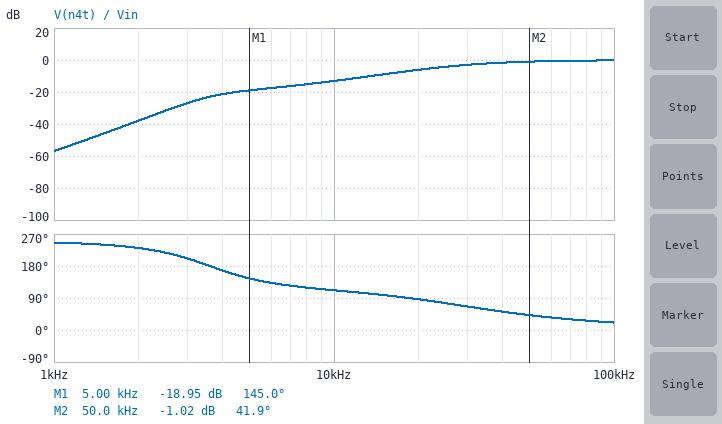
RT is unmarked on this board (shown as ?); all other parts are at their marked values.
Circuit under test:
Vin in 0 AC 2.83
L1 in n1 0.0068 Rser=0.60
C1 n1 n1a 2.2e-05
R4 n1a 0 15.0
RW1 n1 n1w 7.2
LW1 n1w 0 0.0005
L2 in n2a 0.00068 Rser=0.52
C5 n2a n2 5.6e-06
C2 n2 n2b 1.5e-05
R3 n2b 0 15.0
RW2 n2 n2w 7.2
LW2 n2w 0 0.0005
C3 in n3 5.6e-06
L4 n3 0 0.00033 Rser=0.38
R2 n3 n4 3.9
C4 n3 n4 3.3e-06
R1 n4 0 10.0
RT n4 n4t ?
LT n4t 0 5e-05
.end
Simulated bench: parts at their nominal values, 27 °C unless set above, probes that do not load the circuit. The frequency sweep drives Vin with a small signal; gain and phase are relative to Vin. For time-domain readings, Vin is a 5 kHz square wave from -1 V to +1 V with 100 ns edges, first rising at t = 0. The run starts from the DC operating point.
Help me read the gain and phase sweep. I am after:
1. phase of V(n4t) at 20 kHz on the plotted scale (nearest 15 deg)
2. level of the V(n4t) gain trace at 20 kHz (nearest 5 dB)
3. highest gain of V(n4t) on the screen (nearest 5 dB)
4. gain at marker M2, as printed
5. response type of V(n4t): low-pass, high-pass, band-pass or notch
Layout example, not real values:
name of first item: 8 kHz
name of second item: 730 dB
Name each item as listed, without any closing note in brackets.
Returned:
phase of V(n4t) at 20 kHz on the plotted scale: 90 deg
level of the V(n4t) gain trace at 20 kHz: -5 dB
highest gain of V(n4t) on the screen: 0 dB
gain at marker M2, as printed: -1.02 dB
response type of V(n4t): low-pass, high-pass, band-pass or notch: high-pass
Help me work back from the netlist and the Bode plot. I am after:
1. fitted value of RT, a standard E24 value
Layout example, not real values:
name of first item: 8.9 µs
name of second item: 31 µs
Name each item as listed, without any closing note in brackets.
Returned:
fitted value of RT, a standard E24 value: 9.1 Ω
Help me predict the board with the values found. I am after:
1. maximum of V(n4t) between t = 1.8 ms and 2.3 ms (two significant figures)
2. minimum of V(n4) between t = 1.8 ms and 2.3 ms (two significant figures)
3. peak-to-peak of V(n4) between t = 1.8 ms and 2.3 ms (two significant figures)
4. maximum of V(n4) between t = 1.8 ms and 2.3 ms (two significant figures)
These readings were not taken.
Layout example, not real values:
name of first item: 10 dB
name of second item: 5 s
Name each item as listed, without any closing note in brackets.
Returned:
maximum of V(n4t) between t = 1.8 ms and 2.3 ms: 2.0 V
minimum of V(n4) between t = 1.8 ms and 2.3 ms: -2.3 V
peak-to-peak of V(n4) between t = 1.8 ms and 2.3 ms: 4.5 V
maximum of V(n4) between t = 1.8 ms and 2.3 ms: 2.3 V
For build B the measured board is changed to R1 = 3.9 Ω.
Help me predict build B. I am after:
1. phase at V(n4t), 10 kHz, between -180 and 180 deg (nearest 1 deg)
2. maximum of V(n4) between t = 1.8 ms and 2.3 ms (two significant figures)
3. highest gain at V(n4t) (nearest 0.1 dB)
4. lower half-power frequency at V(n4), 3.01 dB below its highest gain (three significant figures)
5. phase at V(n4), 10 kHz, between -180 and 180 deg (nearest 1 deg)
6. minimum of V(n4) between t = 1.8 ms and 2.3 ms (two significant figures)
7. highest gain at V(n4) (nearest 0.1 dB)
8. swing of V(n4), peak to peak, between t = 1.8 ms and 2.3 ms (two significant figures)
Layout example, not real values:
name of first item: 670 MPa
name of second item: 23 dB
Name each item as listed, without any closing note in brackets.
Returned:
phase at V(n4t), 10 kHz, between -180 and 180 deg: 120 deg
maximum of V(n4) between t = 1.8 ms and 2.3 ms: 2.1 V
highest gain at V(n4t): 0 dB
lower half-power frequency at V(n4), 3.01 dB below its highest gain: 24.3 kHz
phase at V(n4), 10 kHz, between -180 and 180 deg: 49 deg
minimum of V(n4) between t = 1.8 ms and 2.3 ms: -2.1 V
highest gain at V(n4): 0 dB
swing of V(n4), peak to peak, between t = 1.8 ms and 2.3 ms: 4.3 V
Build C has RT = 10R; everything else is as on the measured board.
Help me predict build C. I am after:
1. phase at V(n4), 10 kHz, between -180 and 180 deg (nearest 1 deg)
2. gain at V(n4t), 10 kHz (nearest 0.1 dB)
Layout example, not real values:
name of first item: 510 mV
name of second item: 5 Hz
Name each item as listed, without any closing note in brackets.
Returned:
phase at V(n4), 10 kHz, between -180 and 180 deg: 39 deg
gain at V(n4t), 10 kHz: -13.7 dB
